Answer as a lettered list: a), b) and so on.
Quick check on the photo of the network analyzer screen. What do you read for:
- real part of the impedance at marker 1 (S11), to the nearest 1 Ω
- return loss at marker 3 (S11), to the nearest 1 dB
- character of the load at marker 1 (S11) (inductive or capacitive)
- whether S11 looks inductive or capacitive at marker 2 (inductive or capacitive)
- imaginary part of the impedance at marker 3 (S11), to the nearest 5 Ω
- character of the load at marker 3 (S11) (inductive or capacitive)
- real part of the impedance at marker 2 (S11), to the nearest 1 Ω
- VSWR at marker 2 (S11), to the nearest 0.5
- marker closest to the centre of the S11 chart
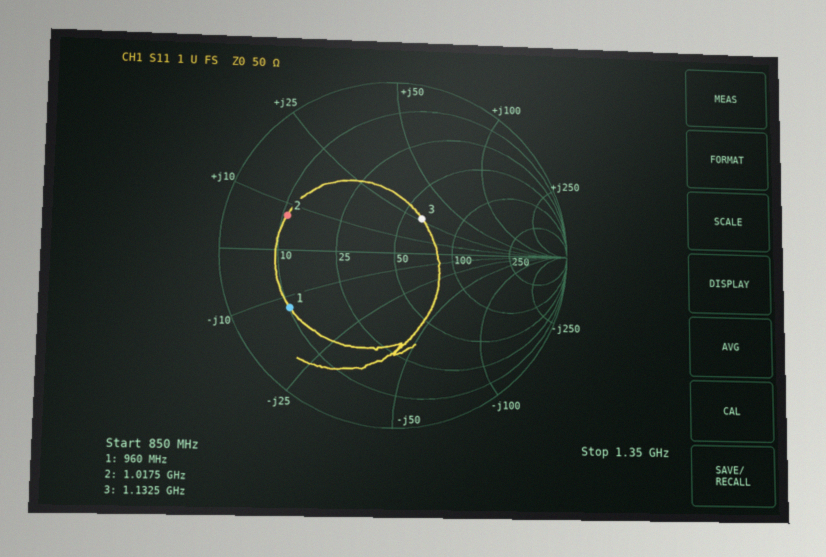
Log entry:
a) 10 Ω
b) 12 dB
c) capacitive
d) inductive
e) +25 Ω
f) inductive
g) 11 Ω
h) 4.5
i) marker 3
